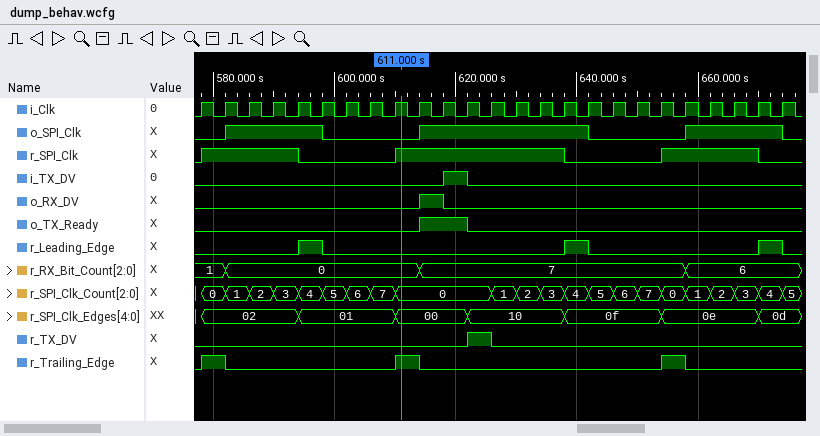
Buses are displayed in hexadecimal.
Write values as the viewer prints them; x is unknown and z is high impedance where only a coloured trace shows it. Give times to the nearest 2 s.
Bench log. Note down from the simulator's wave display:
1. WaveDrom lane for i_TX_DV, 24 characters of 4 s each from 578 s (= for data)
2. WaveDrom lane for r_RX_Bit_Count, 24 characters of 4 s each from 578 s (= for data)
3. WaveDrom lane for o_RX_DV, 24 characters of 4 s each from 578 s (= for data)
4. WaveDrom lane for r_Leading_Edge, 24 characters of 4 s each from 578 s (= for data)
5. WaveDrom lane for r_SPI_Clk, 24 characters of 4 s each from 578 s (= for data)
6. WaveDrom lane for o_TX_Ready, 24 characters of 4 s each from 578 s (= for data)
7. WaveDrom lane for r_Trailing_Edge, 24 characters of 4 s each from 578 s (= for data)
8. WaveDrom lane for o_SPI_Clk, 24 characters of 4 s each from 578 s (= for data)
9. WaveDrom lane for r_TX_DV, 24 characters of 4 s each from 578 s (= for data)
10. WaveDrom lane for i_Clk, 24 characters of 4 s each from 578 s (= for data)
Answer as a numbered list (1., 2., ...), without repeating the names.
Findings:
1. {name: 'i_TX_DV', wave: '0.........10............'}
2. {name: 'r_RX_Bit_Count', wave: '==.......=..........=...', data: '1 0 7 6'}
3. {name: 'o_RX_DV', wave: '0........10.............'}
4. {name: 'r_Leading_Edge', wave: '0...10.........10......1'}
5. {name: 'r_SPI_Clk', wave: '1...0...1......0...1...0'}
6. {name: 'o_TX_Ready', wave: '0........1.0............'}
7. {name: 'r_Trailing_Edge', wave: '10......10.........10...'}
8. {name: 'o_SPI_Clk', wave: '01...0...1......0...1...'}
9. {name: 'r_TX_DV', wave: '0..........10...........'}
10. {name: 'i_Clk', wave: 'p.......................'}
